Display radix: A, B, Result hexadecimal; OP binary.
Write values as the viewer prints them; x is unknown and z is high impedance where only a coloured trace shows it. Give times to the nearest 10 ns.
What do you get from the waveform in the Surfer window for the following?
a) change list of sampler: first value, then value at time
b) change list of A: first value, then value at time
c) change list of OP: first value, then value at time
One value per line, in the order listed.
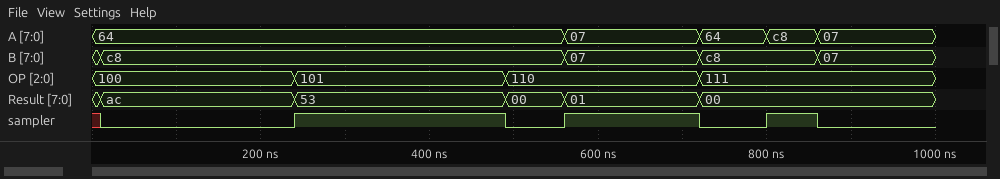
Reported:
x, 0 at 10 ns, 1 at 240 ns, 0 at 490 ns, 1 at 560 ns, 0 at 720 ns, 1 at 800 ns, 0 at 860 ns
64, 07 at 560 ns, 64 at 720 ns, c8 at 800 ns, 07 at 860 ns
100, 101 at 240 ns, 110 at 490 ns, 111 at 720 ns
